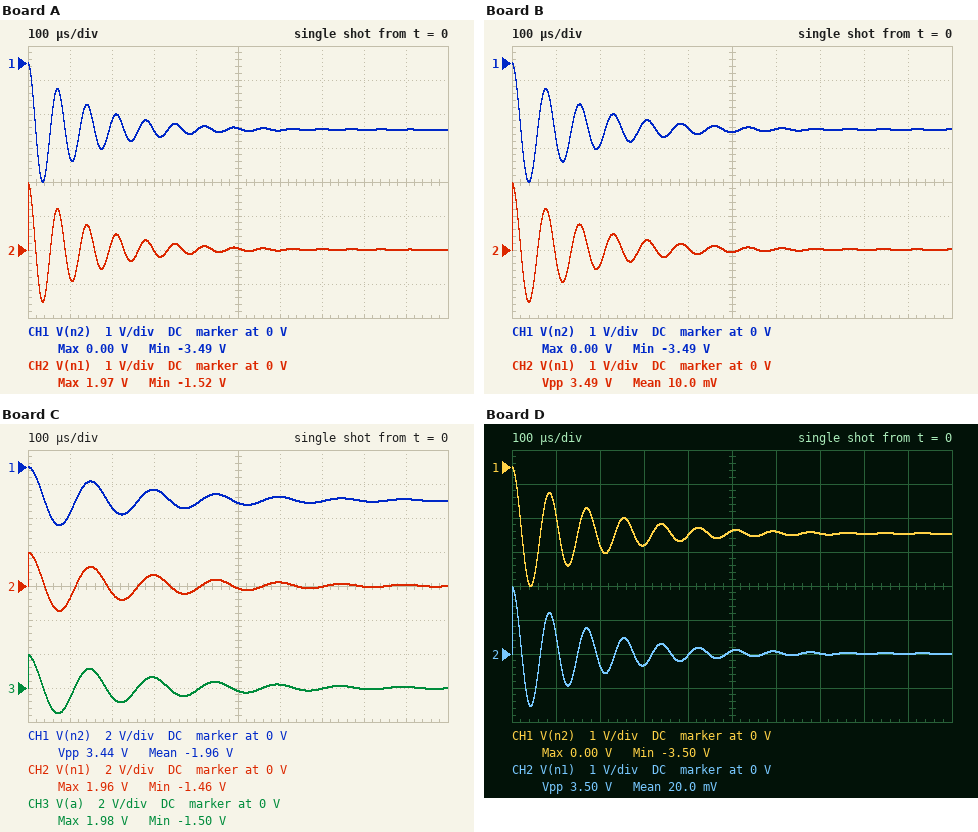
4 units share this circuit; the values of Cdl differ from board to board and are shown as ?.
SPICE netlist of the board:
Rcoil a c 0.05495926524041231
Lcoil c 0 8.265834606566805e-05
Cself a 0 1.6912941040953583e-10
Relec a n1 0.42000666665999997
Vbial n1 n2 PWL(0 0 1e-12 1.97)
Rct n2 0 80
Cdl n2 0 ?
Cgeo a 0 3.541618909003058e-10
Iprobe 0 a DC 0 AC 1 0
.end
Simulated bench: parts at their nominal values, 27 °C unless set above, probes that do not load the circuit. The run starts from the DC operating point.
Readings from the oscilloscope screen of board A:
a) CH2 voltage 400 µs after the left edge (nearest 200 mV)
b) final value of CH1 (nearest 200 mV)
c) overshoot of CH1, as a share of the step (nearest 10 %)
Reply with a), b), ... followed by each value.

a) 0 V
b) -2.0 V
c) 80 %
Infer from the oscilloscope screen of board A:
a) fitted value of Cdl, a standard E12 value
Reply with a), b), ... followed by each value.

a) 1.5 µF
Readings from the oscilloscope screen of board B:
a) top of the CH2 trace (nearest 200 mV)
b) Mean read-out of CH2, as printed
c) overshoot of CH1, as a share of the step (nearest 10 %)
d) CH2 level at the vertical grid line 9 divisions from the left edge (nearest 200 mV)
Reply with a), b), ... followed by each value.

a) 2.0 V
b) 10.0 mV
c) 80 %
d) 0 V
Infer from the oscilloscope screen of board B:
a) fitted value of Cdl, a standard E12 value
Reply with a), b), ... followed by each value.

a) 1.8 µF
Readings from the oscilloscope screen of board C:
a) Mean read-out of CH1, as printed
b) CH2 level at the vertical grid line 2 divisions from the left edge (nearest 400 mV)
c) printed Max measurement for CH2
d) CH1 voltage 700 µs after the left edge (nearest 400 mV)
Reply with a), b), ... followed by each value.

a) -1.96 V
b) -400 mV
c) 1.96 V
d) -2.0 V
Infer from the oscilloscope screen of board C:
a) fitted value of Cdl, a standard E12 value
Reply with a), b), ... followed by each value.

a) 6.8 µF
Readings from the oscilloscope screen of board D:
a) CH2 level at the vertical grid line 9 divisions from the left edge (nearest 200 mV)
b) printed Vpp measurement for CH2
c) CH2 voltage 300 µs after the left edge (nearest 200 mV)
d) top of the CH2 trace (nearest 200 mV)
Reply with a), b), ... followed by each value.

a) 0 V
b) 3.50 V
c) -400 mV
d) 2.0 V
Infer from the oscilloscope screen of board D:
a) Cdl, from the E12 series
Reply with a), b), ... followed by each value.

a) 2.2 µF
